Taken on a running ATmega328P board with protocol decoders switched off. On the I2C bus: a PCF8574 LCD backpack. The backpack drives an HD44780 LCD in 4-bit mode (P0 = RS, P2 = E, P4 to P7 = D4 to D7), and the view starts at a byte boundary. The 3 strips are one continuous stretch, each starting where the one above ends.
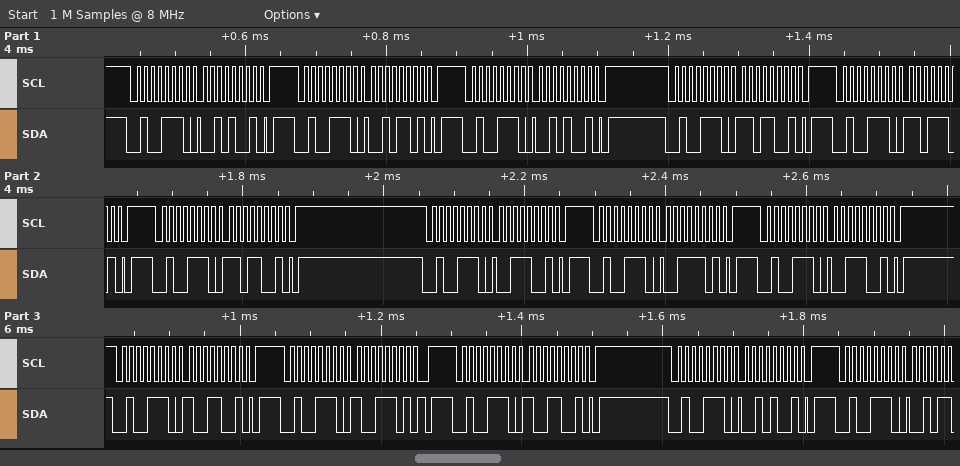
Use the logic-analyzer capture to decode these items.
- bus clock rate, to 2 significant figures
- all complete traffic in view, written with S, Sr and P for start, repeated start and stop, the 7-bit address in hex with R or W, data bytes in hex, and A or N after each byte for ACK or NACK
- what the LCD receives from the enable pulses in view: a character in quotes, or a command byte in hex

100 kHz
S 27W A 29 A P S 27W A 2D A P S 27W A 29 A P S 27W A D9 A P S 27W A DD A P S 27W A D9 A P S 27W A 39 A P S 27W A 3D A P S 27W A 39 A P S 27W A 99 A P S 27W A 9D A P S 27W A 99 A P S 27W A 29 A P S 27W A
'-' '9'
